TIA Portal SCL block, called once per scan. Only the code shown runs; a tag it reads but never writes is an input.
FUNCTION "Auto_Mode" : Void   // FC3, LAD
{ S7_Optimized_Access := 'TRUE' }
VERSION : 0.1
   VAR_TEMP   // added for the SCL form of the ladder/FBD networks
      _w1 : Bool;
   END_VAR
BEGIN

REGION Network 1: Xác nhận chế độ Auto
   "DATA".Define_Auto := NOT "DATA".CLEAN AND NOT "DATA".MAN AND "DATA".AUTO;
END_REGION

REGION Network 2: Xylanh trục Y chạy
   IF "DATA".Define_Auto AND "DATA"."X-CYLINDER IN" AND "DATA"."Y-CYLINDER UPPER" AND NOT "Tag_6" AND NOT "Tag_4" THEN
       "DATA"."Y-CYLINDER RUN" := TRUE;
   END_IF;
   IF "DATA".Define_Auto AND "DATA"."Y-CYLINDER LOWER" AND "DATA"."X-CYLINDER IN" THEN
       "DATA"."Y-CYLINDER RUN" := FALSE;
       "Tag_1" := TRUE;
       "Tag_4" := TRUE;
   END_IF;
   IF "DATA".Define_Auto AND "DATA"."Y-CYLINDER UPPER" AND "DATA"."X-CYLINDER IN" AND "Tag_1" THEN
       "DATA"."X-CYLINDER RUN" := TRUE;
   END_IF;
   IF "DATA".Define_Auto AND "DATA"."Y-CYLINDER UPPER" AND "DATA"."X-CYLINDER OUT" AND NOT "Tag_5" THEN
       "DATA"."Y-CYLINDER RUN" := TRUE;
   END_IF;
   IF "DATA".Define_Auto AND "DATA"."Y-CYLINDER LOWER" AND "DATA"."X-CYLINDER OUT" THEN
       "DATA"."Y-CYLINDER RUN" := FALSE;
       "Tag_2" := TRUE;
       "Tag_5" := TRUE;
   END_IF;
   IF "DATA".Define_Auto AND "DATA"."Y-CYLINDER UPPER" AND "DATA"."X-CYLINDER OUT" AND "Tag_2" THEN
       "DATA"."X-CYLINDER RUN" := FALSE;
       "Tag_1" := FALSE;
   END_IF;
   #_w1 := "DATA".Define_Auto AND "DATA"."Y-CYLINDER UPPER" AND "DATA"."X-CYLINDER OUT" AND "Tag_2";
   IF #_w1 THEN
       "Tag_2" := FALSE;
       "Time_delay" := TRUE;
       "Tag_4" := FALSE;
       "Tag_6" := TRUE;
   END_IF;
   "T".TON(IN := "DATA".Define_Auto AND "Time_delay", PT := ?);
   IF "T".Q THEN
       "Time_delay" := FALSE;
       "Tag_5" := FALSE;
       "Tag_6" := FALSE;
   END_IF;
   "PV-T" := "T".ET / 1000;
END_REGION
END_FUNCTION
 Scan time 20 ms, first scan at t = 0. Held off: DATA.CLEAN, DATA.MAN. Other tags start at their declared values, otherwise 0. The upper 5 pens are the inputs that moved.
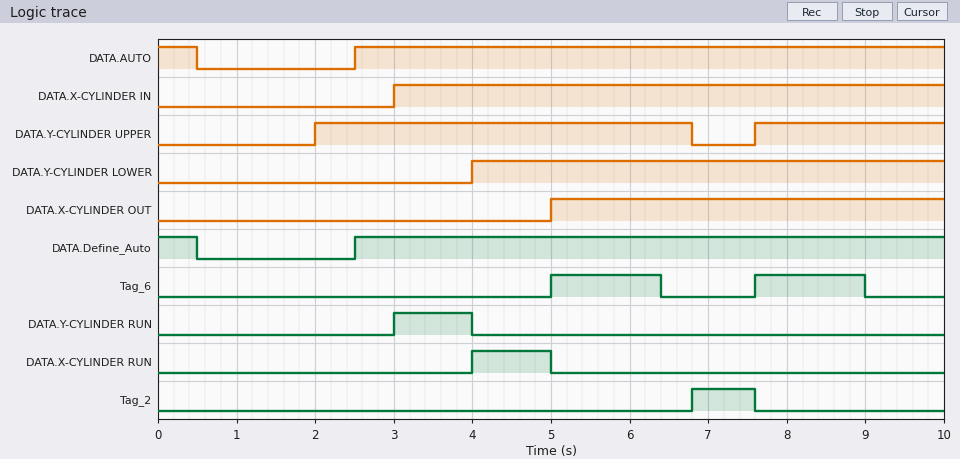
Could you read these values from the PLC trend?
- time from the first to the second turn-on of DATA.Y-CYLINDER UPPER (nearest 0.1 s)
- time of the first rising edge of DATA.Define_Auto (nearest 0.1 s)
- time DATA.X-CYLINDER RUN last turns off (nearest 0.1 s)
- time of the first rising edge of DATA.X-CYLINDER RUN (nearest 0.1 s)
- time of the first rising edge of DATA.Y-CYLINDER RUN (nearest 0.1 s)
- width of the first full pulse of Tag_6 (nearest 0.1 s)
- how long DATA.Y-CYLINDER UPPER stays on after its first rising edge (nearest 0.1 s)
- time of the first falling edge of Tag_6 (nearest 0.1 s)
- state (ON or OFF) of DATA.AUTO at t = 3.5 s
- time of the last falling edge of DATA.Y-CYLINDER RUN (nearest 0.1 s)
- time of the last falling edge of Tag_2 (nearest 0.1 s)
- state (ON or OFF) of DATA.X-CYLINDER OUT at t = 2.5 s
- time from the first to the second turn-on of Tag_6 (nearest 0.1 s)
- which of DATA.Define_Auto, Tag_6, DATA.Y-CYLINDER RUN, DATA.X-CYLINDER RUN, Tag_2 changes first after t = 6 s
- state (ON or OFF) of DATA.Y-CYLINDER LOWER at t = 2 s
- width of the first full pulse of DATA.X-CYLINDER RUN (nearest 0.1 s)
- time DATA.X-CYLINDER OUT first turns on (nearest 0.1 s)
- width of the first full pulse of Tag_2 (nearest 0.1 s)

5.6 s
2.5 s
5.0 s
4.0 s
3.0 s
1.4 s
4.8 s
6.4 s
ON
4.0 s
7.6 s
OFF
2.6 s
Tag_6
OFF
1.0 s
5.0 s
0.8 s
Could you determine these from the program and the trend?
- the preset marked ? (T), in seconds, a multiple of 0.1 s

1.4 s
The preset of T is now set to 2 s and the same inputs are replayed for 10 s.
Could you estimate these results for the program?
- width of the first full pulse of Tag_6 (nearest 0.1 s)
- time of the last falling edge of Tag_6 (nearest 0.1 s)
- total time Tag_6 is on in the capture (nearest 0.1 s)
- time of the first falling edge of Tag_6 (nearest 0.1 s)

2.0 s
9.6 s
4.0 s
7.0 s
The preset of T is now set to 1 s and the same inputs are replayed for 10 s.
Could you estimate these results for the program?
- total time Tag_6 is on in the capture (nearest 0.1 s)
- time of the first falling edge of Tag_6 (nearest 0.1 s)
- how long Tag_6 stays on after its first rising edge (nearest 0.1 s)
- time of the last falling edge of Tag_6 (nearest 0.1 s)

2.0 s
6.0 s
1.0 s
8.6 s
